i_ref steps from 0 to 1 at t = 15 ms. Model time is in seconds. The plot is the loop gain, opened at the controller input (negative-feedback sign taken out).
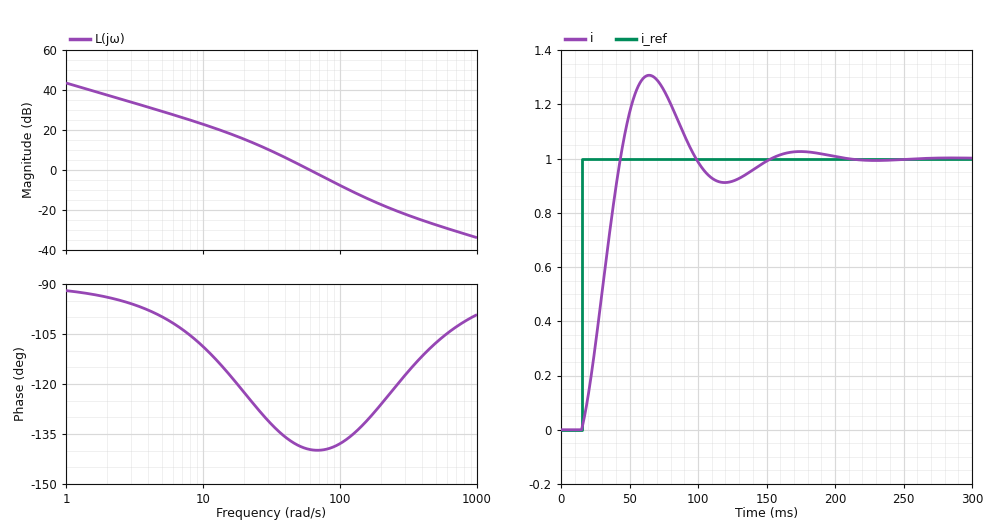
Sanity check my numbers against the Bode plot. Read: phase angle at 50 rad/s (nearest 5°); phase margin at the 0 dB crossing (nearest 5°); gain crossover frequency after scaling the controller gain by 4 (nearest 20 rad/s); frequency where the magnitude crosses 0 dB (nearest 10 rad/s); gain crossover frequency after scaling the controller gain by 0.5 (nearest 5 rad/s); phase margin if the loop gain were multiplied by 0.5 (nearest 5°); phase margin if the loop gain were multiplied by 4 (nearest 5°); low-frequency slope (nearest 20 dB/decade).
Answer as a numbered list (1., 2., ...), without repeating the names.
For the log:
1. -140°
2. 40°
3. 140 rad/s
4. 60 rad/s
5. 40 rad/s
6. 45°
7. 45°
8. -20 dB/decade
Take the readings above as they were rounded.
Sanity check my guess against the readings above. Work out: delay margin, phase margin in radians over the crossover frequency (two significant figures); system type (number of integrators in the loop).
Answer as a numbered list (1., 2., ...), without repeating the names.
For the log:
1. 0.012 s
2. 1
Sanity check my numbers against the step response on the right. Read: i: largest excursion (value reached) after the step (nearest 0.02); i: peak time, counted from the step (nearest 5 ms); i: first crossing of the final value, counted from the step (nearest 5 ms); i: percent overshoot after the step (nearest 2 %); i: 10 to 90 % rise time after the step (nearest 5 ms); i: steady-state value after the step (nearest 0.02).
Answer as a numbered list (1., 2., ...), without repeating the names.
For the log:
1. 1.30
2. 50 ms
3. 30 ms
4. 30 %
5. 20 ms
6. 1.00
